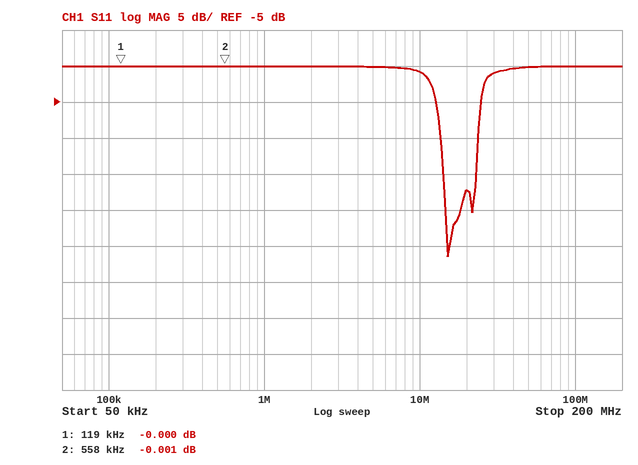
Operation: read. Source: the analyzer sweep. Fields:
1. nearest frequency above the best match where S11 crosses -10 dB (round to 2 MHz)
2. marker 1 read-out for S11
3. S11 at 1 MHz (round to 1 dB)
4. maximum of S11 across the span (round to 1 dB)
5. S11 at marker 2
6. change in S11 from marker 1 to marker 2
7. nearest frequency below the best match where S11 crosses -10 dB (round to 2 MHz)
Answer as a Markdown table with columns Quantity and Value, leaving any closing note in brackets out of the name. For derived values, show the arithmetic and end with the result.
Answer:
| Quantity | Value |
|---|---|
| nearest frequency above the best match where S11 crosses -10 dB | 24 MHz |
| marker 1 read-out for S11 | -0.000 dB |
| S11 at 1 MHz | 0 dB |
| maximum of S11 across the span | 0 dB |
| S11 at marker 2 | -0.001 dB |
| change in S11 from marker 1 to marker 2 | -0.001 − (-0) = -0.001 dB |
| nearest frequency below the best match where S11 crosses -10 dB | 14 MHz |
